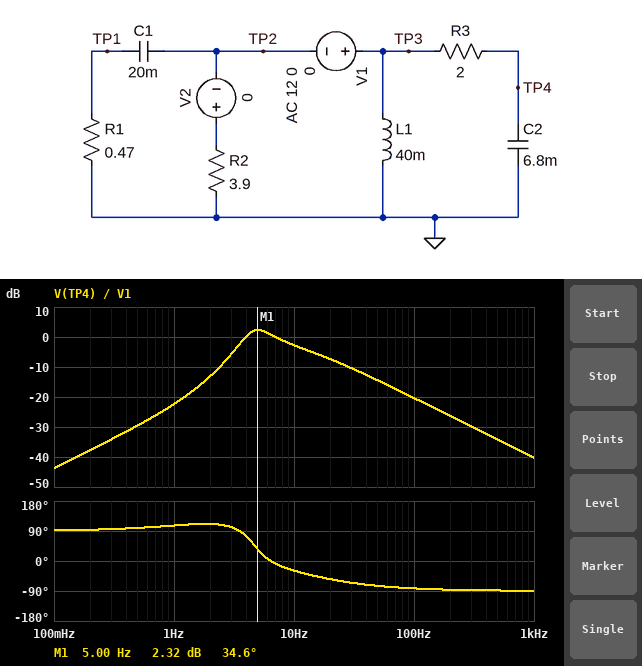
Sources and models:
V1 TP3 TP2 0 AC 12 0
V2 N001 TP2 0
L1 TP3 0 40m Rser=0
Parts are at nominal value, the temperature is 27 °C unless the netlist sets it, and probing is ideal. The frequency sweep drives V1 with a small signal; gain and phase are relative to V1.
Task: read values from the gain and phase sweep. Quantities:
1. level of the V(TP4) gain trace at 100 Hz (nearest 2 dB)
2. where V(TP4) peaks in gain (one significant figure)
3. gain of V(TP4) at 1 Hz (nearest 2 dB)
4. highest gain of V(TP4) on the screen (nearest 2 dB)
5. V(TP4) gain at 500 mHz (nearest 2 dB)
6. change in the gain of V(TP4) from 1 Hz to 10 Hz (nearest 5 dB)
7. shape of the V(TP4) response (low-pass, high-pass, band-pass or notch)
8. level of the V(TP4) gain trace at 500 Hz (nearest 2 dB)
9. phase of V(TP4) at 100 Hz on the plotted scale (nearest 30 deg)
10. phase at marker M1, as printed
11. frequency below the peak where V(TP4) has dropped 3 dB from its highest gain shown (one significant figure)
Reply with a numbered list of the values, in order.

1. -20 dB
2. 5 Hz
3. -22 dB
4. 2 dB
5. -30 dB
6. 20 dB
7. band-pass
8. -34 dB
9. -90 deg
10. 34.6 deg
11. 4 Hz
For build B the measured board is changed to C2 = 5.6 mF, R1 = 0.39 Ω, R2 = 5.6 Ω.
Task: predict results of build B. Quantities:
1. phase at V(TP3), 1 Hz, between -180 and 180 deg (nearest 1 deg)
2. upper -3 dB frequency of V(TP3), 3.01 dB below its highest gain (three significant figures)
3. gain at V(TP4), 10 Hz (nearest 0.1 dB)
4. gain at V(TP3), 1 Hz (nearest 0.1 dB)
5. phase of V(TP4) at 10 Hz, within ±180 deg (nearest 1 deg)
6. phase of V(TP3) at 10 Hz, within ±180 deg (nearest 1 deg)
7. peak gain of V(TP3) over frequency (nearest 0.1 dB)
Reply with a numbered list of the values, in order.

1. 121 deg
2. 7.35 Hz
3. -1.6 dB
4. -24.7 dB
5. -24 deg
6. 11 deg
7. 5.0 dB
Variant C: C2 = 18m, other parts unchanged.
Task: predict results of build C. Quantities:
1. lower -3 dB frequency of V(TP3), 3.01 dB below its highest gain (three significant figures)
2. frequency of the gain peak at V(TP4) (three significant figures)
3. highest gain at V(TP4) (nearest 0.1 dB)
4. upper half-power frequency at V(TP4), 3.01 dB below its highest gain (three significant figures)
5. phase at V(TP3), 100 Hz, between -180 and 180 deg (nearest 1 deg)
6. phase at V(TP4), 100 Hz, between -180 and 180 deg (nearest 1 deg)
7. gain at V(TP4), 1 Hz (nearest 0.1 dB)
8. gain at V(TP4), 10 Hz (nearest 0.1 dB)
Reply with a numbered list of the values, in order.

1. 3.39 Hz
2. 4.38 Hz
3. -3.1 dB
4. 7.00 Hz
5. 2 deg
6. -86 deg
7. -22.4 dB
8. -9.1 dB
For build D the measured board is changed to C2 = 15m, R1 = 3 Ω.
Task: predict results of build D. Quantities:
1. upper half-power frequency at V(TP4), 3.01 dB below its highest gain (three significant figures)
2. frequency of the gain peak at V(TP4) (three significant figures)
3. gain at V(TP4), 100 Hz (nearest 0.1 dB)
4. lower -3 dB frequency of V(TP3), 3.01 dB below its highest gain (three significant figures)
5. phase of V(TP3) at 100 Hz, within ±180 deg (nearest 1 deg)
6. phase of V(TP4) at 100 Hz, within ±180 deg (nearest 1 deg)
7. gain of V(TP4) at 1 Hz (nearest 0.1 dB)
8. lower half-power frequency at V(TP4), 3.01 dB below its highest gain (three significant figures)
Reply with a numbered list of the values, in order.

1. 8.39 Hz
2. 4.47 Hz
3. -30.8 dB
4. 3.11 Hz
5. 1 deg
6. -86 deg
7. -21.7 dB
8. 2.66 Hz
